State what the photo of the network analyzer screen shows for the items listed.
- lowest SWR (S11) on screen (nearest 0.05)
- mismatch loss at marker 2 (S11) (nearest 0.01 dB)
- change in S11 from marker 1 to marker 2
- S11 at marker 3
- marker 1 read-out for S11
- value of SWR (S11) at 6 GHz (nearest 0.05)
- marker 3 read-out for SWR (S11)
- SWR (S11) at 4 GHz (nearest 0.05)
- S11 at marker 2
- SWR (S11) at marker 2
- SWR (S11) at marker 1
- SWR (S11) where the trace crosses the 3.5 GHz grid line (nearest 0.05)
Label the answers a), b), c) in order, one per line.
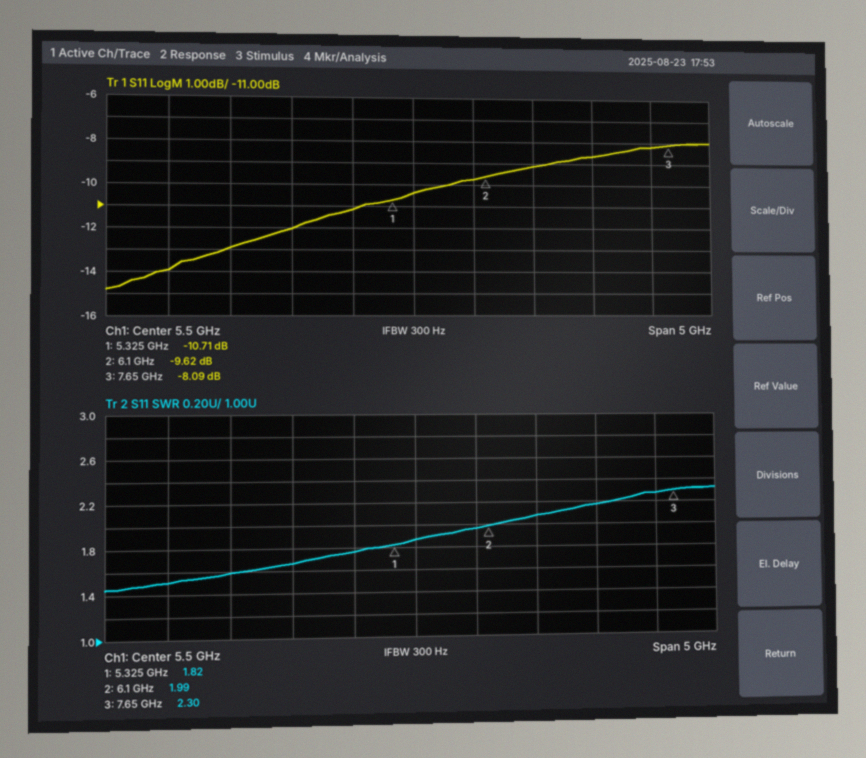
a) 1.45
b) 0.50 dB
c) 1.09 dB
d) -8.09 dB
e) -10.71 dB
f) 1.95
g) 2.30
h) 1.60
i) -9.62 dB
j) 1.99
k) 1.82
l) 1.50
